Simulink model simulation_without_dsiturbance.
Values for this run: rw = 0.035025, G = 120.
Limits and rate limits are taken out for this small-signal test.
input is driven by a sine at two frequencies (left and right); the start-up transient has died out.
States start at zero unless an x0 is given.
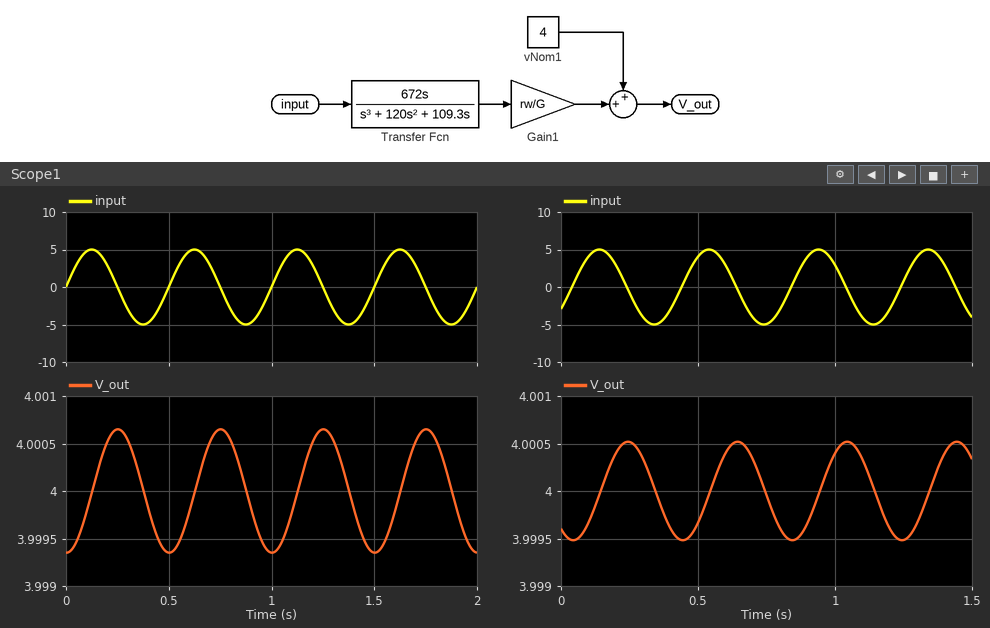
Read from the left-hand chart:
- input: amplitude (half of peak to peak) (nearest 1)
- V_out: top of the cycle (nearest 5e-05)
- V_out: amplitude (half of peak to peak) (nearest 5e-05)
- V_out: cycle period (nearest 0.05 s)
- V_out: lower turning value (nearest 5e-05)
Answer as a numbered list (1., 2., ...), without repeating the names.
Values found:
1. 5
2. 4.00065
3. 0.00065
4. 0.50 s
5. 3.99935
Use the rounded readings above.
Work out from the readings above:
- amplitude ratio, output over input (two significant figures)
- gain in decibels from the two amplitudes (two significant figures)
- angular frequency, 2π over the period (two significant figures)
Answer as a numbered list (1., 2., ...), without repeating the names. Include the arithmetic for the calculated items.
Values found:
1. 0.00065 / 5 = 0.00013
2. 20 log10(0.00065 / 5) = -78 dB
3. 2π / 0.5 = 13 rad/s
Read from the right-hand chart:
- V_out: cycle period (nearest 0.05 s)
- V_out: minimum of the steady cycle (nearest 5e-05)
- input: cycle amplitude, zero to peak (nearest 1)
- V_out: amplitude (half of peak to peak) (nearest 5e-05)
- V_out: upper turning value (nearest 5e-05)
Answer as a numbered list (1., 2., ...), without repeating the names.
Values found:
1. 0.40 s
2. 3.99950
3. 5
4. 0.00050
5. 4.00050
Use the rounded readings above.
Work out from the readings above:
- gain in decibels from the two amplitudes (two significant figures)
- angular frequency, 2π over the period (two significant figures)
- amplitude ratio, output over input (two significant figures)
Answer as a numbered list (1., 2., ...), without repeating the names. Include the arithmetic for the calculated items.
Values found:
1. 20 log10(0.0005 / 5) = -80 dB
2. 2π / 0.4 = 16 rad/s
3. 0.0005 / 5 = 0.00010
